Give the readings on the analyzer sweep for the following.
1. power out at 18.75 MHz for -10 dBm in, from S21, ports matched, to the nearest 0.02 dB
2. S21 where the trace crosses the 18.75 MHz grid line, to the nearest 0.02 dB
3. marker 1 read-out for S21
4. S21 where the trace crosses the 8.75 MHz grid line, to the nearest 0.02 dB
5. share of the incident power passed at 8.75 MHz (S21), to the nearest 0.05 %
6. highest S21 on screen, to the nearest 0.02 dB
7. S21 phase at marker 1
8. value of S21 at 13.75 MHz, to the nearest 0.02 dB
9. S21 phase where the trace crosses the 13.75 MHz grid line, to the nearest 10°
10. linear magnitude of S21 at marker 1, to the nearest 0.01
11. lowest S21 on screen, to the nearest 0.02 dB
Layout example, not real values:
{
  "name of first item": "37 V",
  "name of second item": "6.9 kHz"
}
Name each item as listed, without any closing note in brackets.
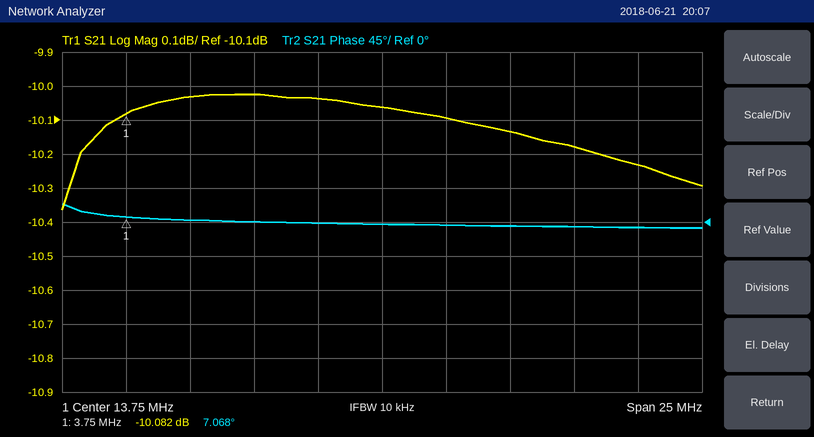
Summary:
{
  "power out at 18.75 MHz for -10 dBm in, from S21, ports matched, to the nearest 0.02 dB": "-20.14 dBm",
  "S21 where the trace crosses the 18.75 MHz grid line, to the nearest 0.02 dB": "-10.14 dB",
  "marker 1 read-out for S21": "-10.082 dB",
  "S21 where the trace crosses the 8.75 MHz grid line, to the nearest 0.02 dB": "-10.02 dB",
  "share of the incident power passed at 8.75 MHz (S21), to the nearest 0.05 %": "9.95 %",
  "highest S21 on screen, to the nearest 0.02 dB": "-10.02 dB",
  "S21 phase at marker 1": "7.068°",
  "value of S21 at 13.75 MHz, to the nearest 0.02 dB": "-10.06 dB",
  "S21 phase where the trace crosses the 13.75 MHz grid line, to the nearest 10°": "0°",
  "linear magnitude of S21 at marker 1, to the nearest 0.01": "0.31",
  "lowest S21 on screen, to the nearest 0.02 dB": "-10.36 dB"
}
